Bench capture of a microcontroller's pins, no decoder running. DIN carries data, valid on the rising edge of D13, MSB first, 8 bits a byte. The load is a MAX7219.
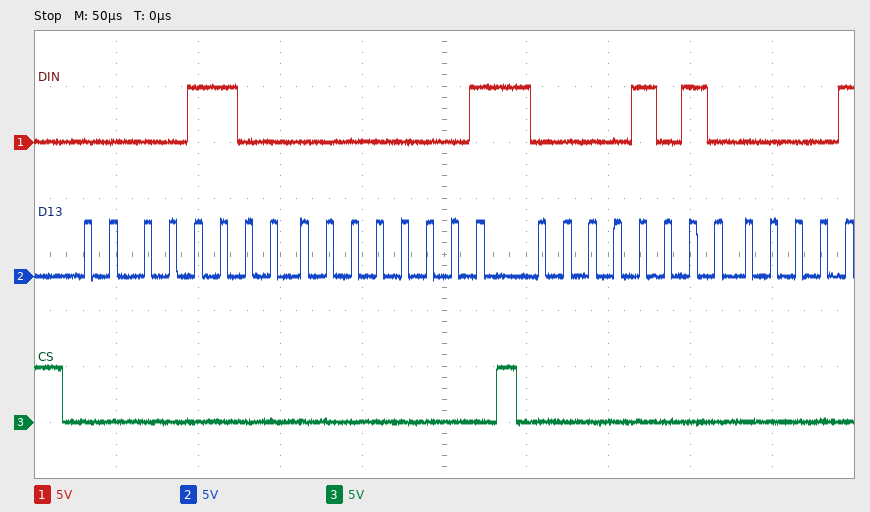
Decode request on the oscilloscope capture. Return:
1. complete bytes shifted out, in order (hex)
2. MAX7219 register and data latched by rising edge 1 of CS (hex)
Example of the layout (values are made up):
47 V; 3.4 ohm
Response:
0x0C 0x01 0x0A; register 0xC, data 0x01
